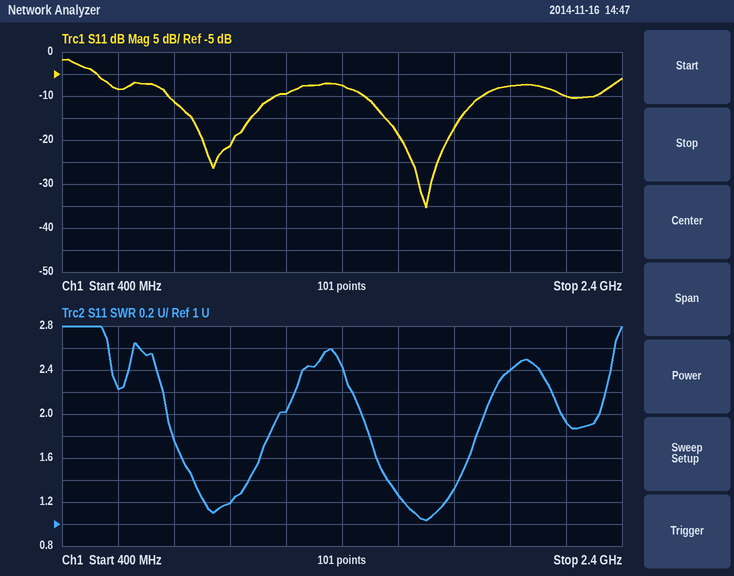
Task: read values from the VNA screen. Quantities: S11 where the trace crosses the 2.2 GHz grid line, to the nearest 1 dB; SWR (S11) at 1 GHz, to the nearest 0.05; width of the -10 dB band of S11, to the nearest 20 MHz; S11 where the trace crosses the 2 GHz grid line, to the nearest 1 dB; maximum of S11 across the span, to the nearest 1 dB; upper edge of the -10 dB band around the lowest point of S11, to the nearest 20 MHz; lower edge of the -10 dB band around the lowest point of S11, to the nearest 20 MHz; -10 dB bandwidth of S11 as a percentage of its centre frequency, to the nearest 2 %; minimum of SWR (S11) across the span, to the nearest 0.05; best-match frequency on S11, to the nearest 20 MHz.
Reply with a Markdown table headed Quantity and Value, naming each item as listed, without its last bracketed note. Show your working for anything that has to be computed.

| Quantity | Value |
|---|---|
| S11 where the trace crosses the 2.2 GHz grid line, to the nearest 1 dB | -10 dB |
| SWR (S11) at 1 GHz, to the nearest 0.05 | 1.20 |
| width of the -10 dB band of S11, to the nearest 20 MHz | 1.90 GHz − 1.48 GHz = 420 MHz |
| S11 where the trace crosses the 2 GHz grid line, to the nearest 1 dB | -8 dB |
| maximum of S11 across the span, to the nearest 1 dB | -2 dB |
| upper edge of the -10 dB band around the lowest point of S11, to the nearest 20 MHz | 1.90 GHz |
| lower edge of the -10 dB band around the lowest point of S11, to the nearest 20 MHz | 1.48 GHz |
| -10 dB bandwidth of S11 as a percentage of its centre frequency, to the nearest 2 % | 420 MHz / 1.69 GHz ≈ 24.9 %, so 24 % to the nearest 2 % |
| minimum of SWR (S11) across the span, to the nearest 0.05 | 1.05 |
| best-match frequency on S11, to the nearest 20 MHz | 1.70 GHz |
